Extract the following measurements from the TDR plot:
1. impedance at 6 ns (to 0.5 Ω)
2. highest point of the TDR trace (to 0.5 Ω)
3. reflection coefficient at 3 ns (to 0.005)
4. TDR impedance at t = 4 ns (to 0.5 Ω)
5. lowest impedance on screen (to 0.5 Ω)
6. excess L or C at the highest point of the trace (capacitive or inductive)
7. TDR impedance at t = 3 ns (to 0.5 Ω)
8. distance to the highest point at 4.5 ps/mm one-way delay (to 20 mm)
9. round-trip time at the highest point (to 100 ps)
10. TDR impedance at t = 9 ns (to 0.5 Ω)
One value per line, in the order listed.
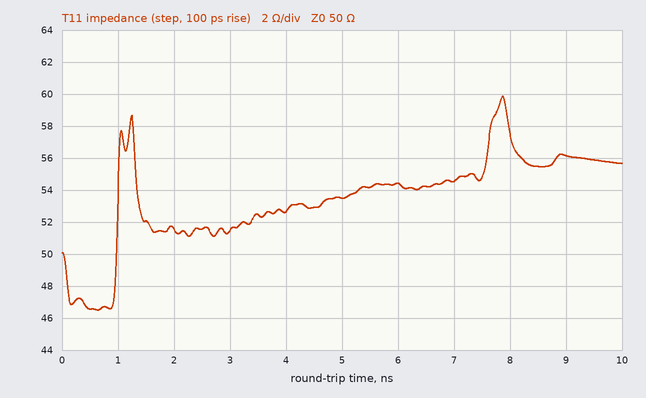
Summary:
54.5 Ω
60.0 Ω
+0.015
52.5 Ω
46.5 Ω
inductive
51.5 Ω
880 mm
7.9 ns
56.0 Ω
